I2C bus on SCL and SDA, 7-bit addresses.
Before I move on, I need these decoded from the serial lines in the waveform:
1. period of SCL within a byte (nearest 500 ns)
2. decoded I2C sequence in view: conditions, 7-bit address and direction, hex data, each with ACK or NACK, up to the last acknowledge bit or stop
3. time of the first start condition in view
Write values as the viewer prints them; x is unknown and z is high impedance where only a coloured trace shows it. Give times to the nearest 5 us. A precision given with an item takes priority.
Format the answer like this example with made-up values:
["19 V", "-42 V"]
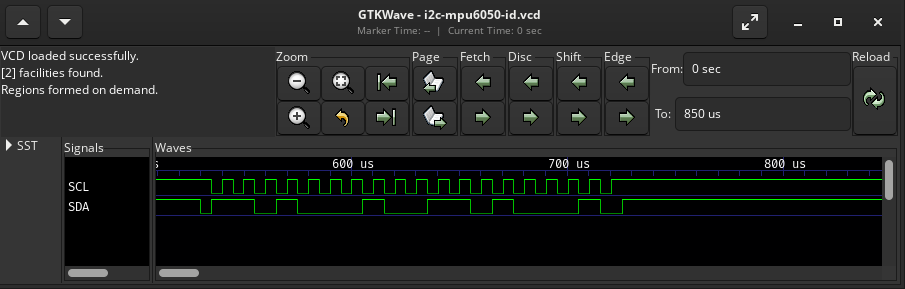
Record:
["10000 ns", "start, address 68 read ACK, 68 NACK, stop", "530 us"]
